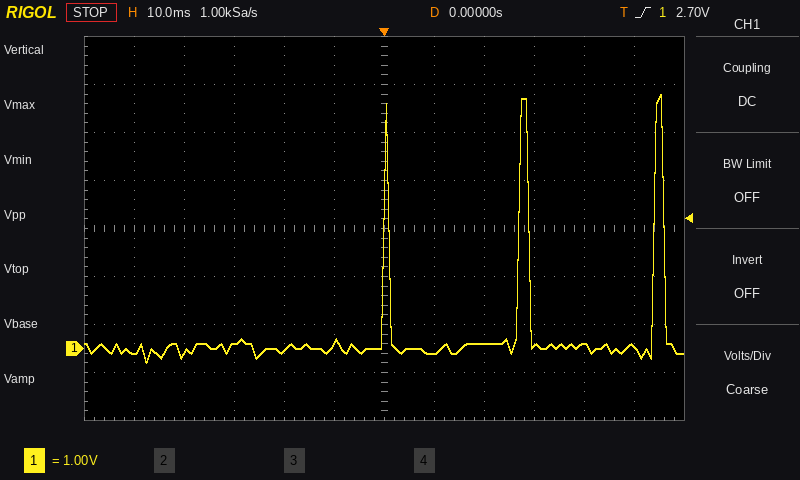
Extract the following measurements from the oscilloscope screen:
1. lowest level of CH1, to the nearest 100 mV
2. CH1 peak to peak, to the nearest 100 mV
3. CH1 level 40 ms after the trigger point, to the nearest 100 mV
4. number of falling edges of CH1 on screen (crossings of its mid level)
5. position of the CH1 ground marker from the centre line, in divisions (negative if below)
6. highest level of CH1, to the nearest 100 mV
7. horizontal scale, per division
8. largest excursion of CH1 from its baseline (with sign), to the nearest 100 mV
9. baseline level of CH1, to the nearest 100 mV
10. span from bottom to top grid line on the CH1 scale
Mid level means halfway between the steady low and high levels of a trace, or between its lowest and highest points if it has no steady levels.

-300 mV
5.6 V
100 mV
3
-2.5 div
5.3 V
10 ms
+5.3 V
0.0 V
8 V
